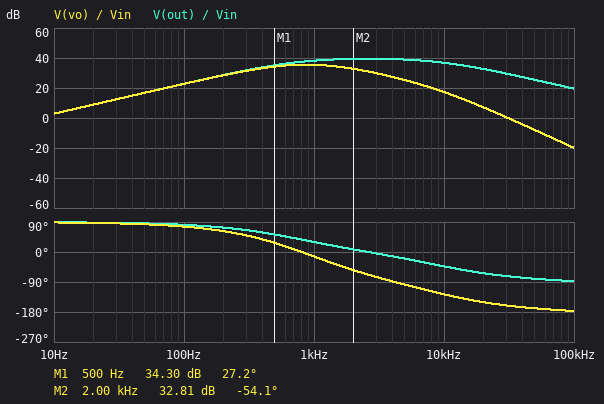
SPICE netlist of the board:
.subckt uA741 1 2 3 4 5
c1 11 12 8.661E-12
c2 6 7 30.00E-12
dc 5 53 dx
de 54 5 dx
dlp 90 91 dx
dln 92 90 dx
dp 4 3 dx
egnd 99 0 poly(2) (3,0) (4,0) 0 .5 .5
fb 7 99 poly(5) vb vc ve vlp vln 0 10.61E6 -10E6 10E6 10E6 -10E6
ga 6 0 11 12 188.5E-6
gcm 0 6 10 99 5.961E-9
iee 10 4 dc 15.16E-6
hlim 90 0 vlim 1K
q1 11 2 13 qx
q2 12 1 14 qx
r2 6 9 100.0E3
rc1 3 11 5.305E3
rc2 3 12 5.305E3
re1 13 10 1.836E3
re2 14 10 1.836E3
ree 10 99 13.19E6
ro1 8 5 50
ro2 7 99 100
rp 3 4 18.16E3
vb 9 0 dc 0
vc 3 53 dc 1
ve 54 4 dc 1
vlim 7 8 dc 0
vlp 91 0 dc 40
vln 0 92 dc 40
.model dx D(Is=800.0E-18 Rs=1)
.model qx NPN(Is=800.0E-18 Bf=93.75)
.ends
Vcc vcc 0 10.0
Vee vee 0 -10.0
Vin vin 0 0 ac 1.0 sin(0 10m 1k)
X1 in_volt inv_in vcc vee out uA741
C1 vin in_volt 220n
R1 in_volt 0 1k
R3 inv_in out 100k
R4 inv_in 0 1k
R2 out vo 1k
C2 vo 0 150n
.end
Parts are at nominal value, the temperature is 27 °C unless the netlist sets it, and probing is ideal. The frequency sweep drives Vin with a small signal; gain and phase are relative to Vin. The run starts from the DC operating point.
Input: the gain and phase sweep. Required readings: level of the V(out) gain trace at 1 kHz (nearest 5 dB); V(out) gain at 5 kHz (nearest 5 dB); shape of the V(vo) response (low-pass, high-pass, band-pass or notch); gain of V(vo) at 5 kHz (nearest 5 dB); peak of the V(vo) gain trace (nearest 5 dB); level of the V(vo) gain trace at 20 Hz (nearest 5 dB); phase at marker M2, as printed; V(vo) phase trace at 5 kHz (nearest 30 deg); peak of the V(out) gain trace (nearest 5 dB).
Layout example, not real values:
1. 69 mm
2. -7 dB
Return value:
1. 40 dB
2. 40 dB
3. band-pass
4. 25 dB
5. 35 dB
6. 10 dB
7. -54.1 deg
8. -90 deg
9. 40 dB
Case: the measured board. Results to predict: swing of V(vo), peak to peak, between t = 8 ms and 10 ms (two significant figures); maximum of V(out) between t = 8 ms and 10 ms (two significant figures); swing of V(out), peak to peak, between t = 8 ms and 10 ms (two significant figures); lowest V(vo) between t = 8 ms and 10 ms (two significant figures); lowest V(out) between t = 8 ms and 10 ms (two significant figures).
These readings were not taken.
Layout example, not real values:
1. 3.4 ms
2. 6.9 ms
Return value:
1. 1.2 V
2. 820 mV
3. 1.6 V
4. -590 mV
5. -810 mV
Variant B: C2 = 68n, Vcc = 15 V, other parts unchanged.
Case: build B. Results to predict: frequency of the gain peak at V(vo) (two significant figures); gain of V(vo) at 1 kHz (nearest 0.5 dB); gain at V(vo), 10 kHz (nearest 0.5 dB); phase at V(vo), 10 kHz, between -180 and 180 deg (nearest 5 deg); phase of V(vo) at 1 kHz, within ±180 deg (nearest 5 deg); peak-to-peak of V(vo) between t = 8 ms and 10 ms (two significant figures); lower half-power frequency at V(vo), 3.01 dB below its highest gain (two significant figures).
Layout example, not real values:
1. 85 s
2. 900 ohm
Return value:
1. 1.3 kHz
2. 37.5 dB
3. 24.0 dB
4. -120 deg
5. 5 deg
6. 1.5 V
7. 470 Hz
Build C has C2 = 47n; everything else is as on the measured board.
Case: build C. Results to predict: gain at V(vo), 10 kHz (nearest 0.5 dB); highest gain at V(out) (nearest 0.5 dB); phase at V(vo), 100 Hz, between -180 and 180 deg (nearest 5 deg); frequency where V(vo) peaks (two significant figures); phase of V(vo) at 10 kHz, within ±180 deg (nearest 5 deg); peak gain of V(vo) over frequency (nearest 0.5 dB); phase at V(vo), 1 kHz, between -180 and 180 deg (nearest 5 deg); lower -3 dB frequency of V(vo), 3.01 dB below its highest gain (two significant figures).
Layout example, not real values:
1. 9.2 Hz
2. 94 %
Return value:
1. 27.0 dB
2. 39.5 dB
3. 80 deg
4. 1.5 kHz
5. -115 deg
6. 38.5 dB
7. 15 deg
8. 520 Hz
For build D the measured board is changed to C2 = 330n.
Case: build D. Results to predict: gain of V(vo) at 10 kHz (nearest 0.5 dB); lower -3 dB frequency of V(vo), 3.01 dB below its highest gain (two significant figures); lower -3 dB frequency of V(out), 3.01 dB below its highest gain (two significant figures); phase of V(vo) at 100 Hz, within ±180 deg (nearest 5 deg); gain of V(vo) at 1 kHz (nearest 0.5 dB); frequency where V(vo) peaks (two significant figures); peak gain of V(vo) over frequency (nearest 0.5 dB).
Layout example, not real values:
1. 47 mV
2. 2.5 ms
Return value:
1. 10.5 dB
2. 240 Hz
3. 630 Hz
4. 70 deg
5. 31.0 dB
6. 590 Hz
7. 32.0 dB
